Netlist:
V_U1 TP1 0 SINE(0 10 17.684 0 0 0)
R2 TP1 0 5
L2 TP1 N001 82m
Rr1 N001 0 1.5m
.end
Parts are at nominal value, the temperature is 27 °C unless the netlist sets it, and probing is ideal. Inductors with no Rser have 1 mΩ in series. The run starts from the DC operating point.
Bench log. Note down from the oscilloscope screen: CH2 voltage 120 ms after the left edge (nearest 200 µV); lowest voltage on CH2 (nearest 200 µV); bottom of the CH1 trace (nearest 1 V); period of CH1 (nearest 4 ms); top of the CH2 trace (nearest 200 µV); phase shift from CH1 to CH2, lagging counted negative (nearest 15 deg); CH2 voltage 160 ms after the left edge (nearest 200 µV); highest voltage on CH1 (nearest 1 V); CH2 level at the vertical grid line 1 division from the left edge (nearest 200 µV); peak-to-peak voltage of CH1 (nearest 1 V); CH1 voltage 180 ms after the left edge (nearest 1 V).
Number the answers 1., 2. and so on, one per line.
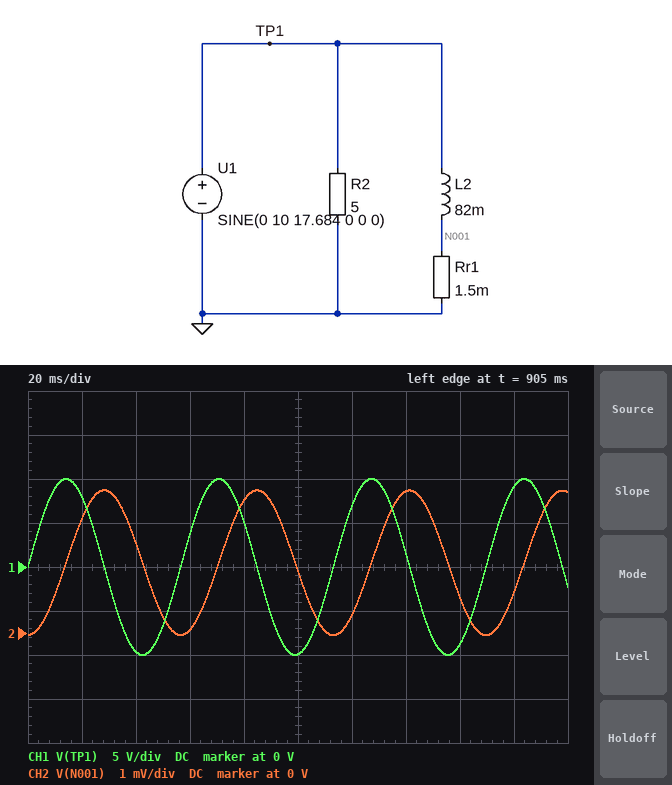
1. 400 µV
2. 0 V
3. -10 V
4. 56 ms
5. 3.2 mV
6. -90 deg
7. 800 µV
8. 10 V
9. 2.6 mV
10. 20 V
11. 9 V
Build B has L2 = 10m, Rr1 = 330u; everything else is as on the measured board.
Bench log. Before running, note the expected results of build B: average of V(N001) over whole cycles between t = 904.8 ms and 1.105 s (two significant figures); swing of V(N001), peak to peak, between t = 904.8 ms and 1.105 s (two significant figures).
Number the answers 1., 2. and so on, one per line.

1. 2.6 mV
2. 6.0 mV
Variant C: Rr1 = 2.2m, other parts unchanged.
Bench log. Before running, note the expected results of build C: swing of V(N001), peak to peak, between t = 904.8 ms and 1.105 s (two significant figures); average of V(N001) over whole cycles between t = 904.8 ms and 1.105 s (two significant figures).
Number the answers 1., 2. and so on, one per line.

1. 4.8 mV
2. 2.3 mV
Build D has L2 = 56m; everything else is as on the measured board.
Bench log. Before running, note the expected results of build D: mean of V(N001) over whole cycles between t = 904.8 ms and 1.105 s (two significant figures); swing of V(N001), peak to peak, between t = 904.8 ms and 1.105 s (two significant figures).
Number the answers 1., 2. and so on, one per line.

1. 2.3 mV
2. 4.8 mV
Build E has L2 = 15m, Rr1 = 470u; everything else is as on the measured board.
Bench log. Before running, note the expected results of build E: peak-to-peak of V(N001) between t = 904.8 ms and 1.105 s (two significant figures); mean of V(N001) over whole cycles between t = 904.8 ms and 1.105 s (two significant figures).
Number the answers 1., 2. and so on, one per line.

1. 5.7 mV
2. 2.6 mV
